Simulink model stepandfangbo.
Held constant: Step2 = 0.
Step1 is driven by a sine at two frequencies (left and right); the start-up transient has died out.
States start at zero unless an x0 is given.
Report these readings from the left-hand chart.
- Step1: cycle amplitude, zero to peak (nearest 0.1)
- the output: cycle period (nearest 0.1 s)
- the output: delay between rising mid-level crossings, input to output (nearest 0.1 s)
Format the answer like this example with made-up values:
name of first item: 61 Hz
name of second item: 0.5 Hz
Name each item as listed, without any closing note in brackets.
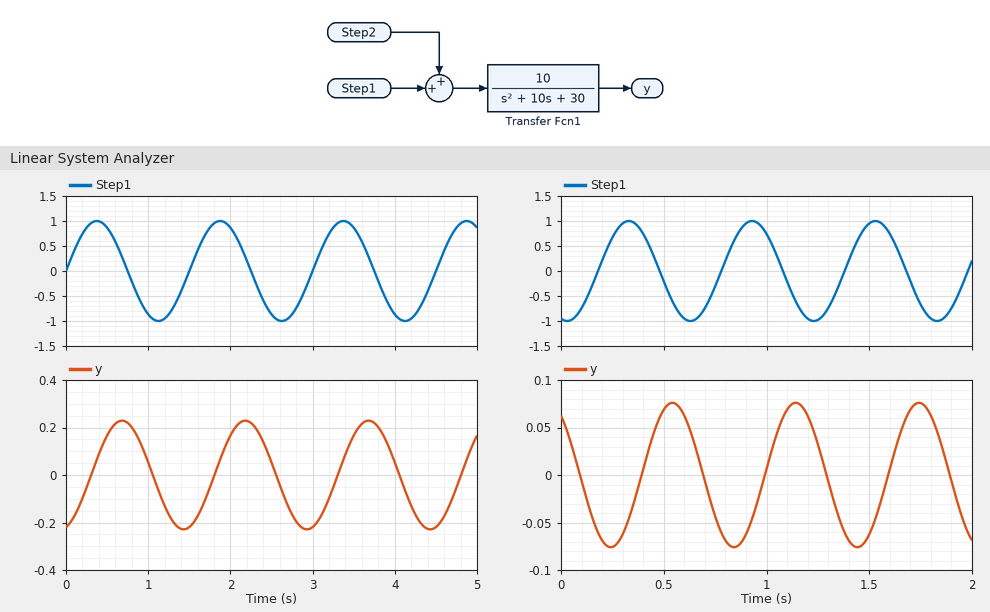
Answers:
Step1: cycle amplitude, zero to peak: 1.0
the output: cycle period: 1.5 s
the output: delay between rising mid-level crossings, input to output: 0.3 s
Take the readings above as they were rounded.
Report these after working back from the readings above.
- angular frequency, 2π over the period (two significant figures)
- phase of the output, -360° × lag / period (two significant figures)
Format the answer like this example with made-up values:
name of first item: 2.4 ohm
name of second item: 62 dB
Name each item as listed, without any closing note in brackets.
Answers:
angular frequency, 2π over the period: 4.2 rad/s
phase of the output, -360° × lag / period: -72°
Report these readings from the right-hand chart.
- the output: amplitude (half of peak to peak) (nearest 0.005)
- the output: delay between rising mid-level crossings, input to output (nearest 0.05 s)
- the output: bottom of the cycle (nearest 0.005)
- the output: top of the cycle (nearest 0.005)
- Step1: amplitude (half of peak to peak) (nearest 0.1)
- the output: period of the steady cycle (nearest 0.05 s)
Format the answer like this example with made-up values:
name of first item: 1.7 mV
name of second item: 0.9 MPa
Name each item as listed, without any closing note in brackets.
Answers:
the output: amplitude (half of peak to peak): 0.075
the output: delay between rising mid-level crossings, input to output: 0.20 s
the output: bottom of the cycle: -0.075
the output: top of the cycle: 0.075
Step1: amplitude (half of peak to peak): 1.0
the output: period of the steady cycle: 0.60 s
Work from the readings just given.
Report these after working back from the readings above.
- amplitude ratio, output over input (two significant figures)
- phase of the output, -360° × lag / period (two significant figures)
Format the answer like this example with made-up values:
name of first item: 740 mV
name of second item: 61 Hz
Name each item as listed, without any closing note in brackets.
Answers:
amplitude ratio, output over input: 0.075
phase of the output, -360° × lag / period: -120°
